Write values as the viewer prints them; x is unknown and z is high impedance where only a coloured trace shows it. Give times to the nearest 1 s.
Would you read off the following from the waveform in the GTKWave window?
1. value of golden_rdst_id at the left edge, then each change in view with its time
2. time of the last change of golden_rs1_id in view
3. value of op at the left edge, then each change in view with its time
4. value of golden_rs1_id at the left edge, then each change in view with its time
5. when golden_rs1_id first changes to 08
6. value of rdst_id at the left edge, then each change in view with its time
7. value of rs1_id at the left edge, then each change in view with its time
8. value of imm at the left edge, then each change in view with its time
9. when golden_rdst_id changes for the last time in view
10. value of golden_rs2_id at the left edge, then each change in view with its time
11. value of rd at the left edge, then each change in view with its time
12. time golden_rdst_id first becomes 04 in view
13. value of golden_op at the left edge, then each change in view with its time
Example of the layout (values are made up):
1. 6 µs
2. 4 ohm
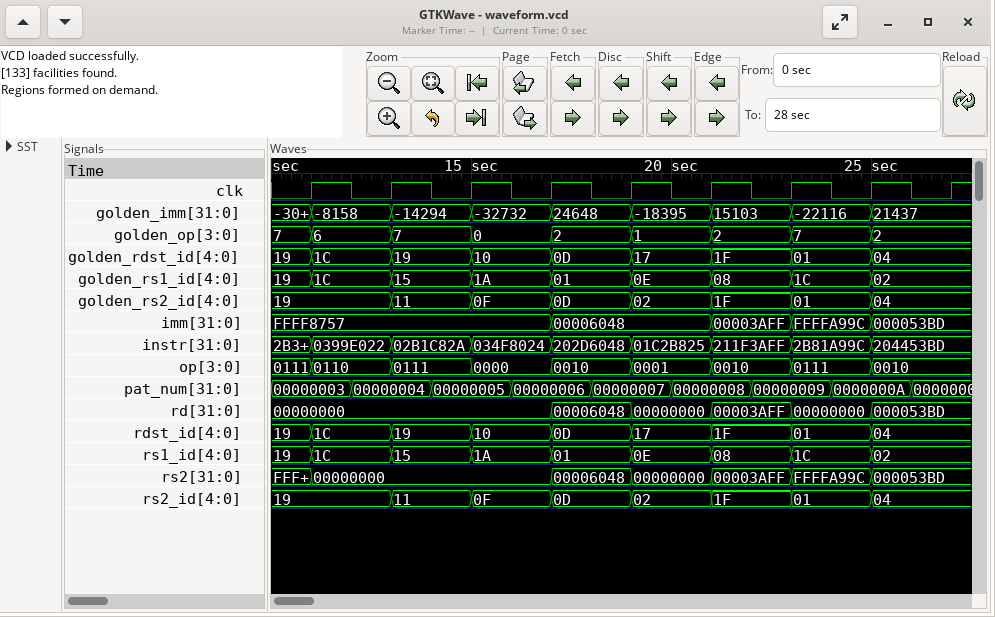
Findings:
1. 19, 1C at 11 s, 19 at 13 s, 10 at 15 s, 0D at 17 s, 17 at 19 s, 1F at 21 s, 01 at 23 s, 04 at 25 s
2. 25 s
3. 0111, 0110 at 11 s, 0111 at 13 s, 0000 at 15 s, 0010 at 17 s, 0001 at 19 s, 0010 at 21 s, 0111 at 23 s, 0010 at 25 s
4. 19, 1C at 11 s, 15 at 13 s, 1A at 15 s, 01 at 17 s, 0E at 19 s, 08 at 21 s, 1C at 23 s, 02 at 25 s
5. 21 s
6. 19, 1C at 11 s, 19 at 13 s, 10 at 15 s, 0D at 17 s, 17 at 19 s, 1F at 21 s, 01 at 23 s, 04 at 25 s
7. 19, 1C at 11 s, 15 at 13 s, 1A at 15 s, 01 at 17 s, 0E at 19 s, 08 at 21 s, 1C at 23 s, 02 at 25 s
8. FFFF8757, 00006048 at 17 s, 00003AFF at 21 s, FFFFA99C at 23 s, 000053BD at 25 s
9. 25 s
10. 19, 11 at 13 s, 0F at 15 s, 0D at 17 s, 02 at 19 s, 1F at 21 s, 01 at 23 s, 04 at 25 s
11. 00000000, 00006048 at 17 s, 00000000 at 19 s, 00003AFF at 21 s, 00000000 at 23 s, 000053BD at 25 s
12. 25 s
13. 7, 6 at 11 s, 7 at 13 s, 0 at 15 s, 2 at 17 s, 1 at 19 s, 2 at 21 s, 7 at 23 s, 2 at 25 s
